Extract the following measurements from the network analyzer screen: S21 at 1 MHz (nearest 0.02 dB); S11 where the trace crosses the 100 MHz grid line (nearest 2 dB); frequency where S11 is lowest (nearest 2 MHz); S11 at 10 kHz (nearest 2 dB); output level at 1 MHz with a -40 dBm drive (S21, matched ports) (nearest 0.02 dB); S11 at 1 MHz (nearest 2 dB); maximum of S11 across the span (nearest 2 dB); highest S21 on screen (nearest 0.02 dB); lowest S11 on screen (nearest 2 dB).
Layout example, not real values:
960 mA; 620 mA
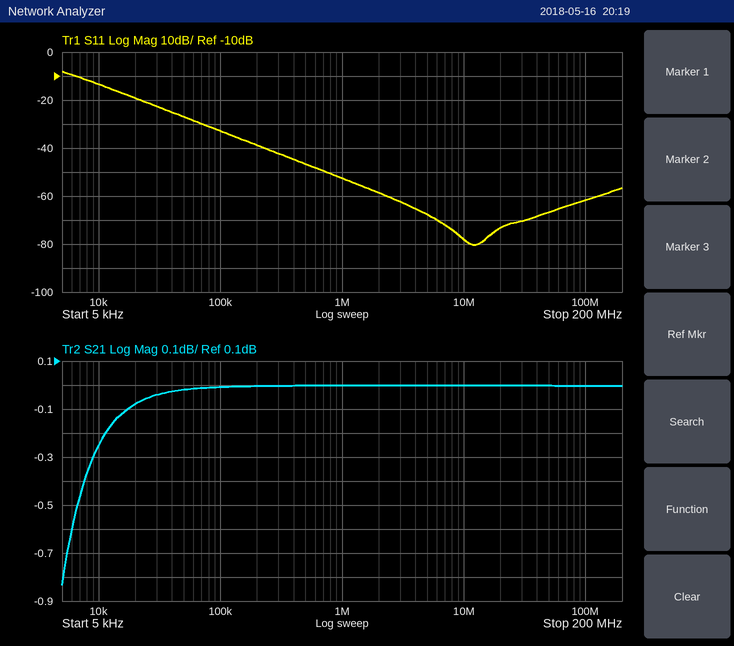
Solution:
0.00 dB; -62 dB; 12 MHz; -14 dB; -40.00 dBm; -52 dB; -8 dB; 0.00 dB; -80 dB
